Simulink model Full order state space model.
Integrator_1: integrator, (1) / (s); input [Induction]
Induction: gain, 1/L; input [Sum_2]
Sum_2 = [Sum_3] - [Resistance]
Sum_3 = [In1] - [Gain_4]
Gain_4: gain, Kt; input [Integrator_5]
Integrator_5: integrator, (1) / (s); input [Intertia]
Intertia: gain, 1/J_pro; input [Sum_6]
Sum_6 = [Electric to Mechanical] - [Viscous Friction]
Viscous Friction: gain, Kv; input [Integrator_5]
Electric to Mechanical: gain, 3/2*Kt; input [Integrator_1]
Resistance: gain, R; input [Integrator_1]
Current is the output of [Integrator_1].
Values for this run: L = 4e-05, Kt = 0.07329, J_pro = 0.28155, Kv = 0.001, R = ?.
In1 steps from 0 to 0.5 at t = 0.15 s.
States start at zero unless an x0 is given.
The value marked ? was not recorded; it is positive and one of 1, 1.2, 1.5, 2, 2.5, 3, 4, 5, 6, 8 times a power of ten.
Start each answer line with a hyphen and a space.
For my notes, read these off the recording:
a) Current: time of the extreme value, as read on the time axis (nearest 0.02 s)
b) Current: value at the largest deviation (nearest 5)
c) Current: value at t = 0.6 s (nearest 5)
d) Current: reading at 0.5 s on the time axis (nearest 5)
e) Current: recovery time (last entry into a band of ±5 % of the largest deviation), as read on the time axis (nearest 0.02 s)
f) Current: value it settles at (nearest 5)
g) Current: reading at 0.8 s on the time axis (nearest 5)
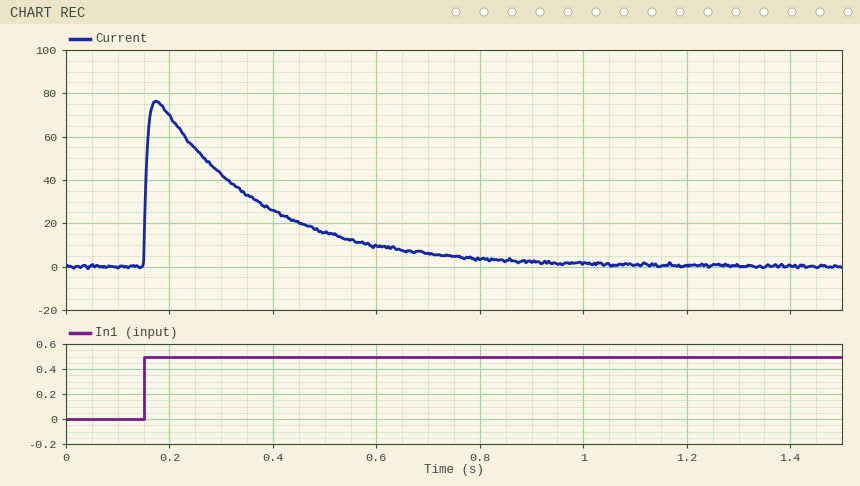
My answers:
- 0.18 s
- 75
- 10
- 15
- 0.78 s
- 0
- 5
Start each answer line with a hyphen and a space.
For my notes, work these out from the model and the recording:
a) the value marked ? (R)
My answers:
- 0.006
